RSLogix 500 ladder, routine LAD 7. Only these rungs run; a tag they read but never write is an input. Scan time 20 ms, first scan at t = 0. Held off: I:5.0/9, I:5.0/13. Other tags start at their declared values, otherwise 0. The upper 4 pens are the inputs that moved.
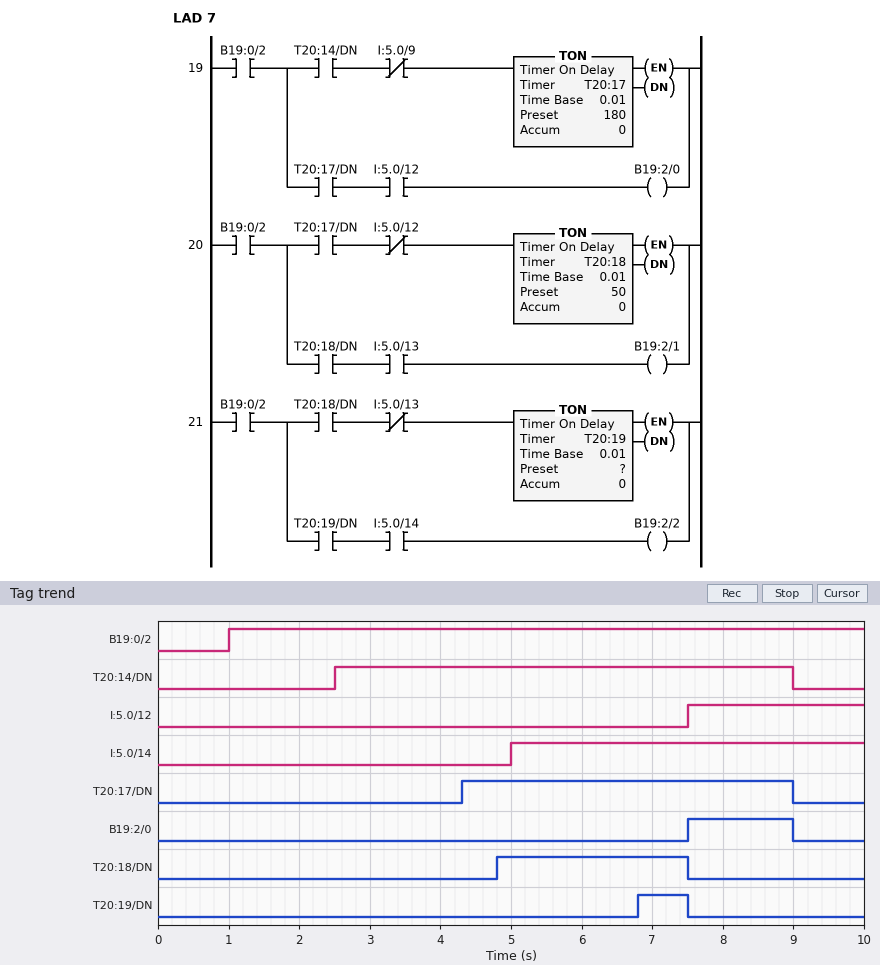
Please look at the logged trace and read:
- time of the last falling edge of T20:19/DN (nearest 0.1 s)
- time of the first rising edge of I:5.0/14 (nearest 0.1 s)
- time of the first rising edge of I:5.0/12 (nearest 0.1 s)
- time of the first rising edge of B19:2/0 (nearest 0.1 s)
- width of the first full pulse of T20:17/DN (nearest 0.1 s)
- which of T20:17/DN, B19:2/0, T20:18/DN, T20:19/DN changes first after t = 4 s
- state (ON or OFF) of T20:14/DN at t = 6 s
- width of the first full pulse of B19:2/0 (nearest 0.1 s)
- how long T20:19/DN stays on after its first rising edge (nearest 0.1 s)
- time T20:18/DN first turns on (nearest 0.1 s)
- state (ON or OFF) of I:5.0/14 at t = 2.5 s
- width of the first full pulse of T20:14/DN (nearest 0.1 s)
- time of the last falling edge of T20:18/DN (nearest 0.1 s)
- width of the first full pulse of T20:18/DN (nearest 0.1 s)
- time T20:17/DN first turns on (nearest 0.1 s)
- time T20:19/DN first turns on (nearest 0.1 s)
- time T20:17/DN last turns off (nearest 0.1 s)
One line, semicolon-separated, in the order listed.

7.5 s; 5.0 s; 7.5 s; 7.5 s; 4.7 s; T20:17/DN; ON; 1.5 s; 0.7 s; 4.8 s; OFF; 6.5 s; 7.5 s; 2.7 s; 4.3 s; 6.8 s; 9.0 s
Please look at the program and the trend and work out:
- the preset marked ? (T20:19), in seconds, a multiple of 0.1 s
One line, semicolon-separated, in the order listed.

2.0 s
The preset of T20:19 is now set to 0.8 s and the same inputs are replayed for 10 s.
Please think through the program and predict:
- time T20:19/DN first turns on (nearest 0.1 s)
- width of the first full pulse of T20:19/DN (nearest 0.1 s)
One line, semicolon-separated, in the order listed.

5.6 s; 1.9 s
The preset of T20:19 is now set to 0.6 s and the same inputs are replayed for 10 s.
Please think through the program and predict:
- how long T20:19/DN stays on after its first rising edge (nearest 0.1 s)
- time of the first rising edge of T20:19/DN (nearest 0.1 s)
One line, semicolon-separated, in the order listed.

2.1 s; 5.4 s
